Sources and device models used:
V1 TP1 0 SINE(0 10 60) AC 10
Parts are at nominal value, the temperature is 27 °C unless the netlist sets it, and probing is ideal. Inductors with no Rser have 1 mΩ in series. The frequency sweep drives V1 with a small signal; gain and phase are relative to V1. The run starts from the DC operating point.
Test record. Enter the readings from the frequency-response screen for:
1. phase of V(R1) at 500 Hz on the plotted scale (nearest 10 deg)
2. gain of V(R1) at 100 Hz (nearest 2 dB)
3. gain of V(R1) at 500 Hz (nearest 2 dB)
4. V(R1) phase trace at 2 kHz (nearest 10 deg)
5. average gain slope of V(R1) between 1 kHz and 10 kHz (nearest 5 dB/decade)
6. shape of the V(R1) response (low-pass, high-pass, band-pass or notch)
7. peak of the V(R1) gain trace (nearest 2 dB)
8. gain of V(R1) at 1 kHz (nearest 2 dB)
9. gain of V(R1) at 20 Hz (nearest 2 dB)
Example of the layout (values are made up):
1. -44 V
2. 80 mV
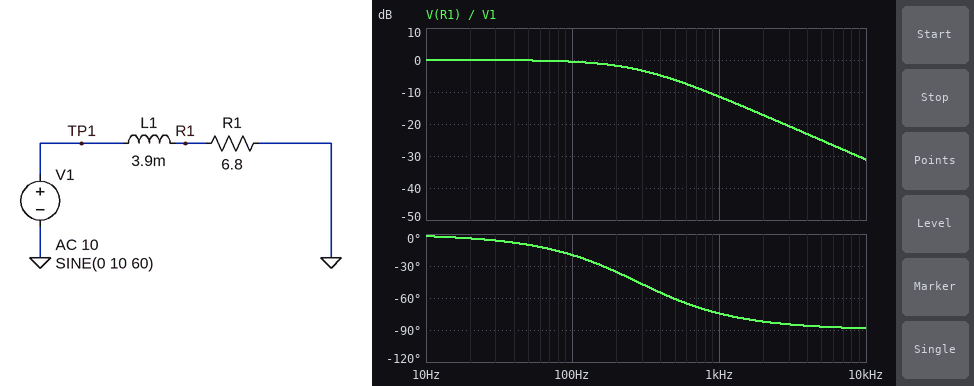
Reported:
1. -60 deg
2. 0 dB
3. -6 dB
4. -80 deg
5. -20 dB/decade
6. low-pass
7. 0 dB
8. -12 dB
9. 0 dB
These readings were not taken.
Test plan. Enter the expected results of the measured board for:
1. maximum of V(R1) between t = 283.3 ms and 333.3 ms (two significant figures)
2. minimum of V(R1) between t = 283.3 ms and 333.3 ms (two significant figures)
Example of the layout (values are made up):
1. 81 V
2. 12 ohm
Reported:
1. 9.8 V
2. -9.8 V
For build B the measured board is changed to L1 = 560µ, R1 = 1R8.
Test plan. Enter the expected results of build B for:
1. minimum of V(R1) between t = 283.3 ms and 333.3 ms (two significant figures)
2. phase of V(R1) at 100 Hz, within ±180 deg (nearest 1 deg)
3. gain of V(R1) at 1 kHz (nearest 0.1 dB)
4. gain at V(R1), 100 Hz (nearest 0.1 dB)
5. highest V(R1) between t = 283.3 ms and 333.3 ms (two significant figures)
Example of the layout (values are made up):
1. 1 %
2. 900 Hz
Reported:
1. -9.9 V
2. -11 deg
3. -6.8 dB
4. -0.2 dB
5. 9.9 V
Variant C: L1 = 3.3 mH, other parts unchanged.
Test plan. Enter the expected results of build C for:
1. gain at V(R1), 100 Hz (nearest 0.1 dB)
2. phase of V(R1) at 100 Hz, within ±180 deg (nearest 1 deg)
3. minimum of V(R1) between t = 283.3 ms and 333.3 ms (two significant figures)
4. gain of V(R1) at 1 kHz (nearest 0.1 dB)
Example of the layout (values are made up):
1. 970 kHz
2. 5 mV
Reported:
1. -0.4 dB
2. -17 deg
3. -9.8 V
4. -10.1 dB
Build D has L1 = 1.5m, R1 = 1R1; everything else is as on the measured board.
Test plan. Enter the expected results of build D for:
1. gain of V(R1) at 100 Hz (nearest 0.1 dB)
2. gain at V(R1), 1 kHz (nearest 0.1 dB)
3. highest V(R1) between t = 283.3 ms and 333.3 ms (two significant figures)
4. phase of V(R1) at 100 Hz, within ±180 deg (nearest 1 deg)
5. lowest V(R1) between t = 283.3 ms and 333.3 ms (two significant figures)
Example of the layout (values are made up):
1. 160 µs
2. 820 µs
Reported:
1. -2.4 dB
2. -18.7 dB
3. 8.9 V
4. -41 deg
5. -8.9 V
